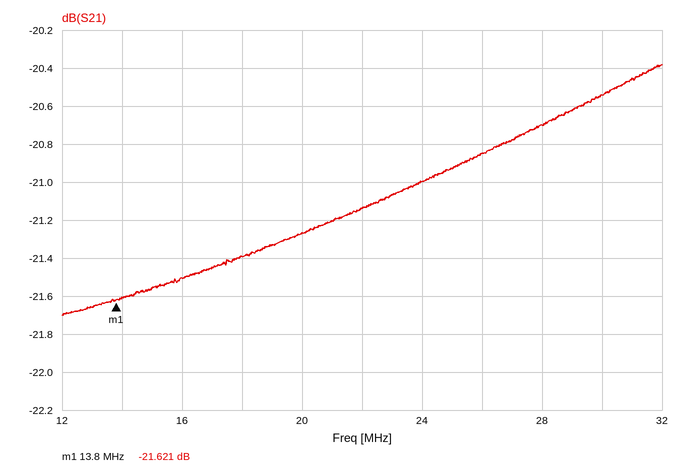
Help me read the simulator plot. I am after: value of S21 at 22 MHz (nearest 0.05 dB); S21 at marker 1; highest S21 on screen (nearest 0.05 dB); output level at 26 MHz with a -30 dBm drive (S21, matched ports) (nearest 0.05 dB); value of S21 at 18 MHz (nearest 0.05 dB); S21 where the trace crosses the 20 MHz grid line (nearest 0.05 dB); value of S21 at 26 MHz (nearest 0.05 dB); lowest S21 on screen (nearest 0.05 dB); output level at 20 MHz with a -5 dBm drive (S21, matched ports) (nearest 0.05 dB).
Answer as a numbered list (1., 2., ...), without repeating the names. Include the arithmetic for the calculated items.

1. -21.15 dB
2. -21.621 dB
3. -20.40 dB
4. -30 dBm + (-20.85 dB) = -50.85 dBm
5. -21.40 dB
6. -21.25 dB
7. -20.85 dB
8. -21.70 dB
9. -5 dBm + (-21.25 dB) = -26.25 dBm
